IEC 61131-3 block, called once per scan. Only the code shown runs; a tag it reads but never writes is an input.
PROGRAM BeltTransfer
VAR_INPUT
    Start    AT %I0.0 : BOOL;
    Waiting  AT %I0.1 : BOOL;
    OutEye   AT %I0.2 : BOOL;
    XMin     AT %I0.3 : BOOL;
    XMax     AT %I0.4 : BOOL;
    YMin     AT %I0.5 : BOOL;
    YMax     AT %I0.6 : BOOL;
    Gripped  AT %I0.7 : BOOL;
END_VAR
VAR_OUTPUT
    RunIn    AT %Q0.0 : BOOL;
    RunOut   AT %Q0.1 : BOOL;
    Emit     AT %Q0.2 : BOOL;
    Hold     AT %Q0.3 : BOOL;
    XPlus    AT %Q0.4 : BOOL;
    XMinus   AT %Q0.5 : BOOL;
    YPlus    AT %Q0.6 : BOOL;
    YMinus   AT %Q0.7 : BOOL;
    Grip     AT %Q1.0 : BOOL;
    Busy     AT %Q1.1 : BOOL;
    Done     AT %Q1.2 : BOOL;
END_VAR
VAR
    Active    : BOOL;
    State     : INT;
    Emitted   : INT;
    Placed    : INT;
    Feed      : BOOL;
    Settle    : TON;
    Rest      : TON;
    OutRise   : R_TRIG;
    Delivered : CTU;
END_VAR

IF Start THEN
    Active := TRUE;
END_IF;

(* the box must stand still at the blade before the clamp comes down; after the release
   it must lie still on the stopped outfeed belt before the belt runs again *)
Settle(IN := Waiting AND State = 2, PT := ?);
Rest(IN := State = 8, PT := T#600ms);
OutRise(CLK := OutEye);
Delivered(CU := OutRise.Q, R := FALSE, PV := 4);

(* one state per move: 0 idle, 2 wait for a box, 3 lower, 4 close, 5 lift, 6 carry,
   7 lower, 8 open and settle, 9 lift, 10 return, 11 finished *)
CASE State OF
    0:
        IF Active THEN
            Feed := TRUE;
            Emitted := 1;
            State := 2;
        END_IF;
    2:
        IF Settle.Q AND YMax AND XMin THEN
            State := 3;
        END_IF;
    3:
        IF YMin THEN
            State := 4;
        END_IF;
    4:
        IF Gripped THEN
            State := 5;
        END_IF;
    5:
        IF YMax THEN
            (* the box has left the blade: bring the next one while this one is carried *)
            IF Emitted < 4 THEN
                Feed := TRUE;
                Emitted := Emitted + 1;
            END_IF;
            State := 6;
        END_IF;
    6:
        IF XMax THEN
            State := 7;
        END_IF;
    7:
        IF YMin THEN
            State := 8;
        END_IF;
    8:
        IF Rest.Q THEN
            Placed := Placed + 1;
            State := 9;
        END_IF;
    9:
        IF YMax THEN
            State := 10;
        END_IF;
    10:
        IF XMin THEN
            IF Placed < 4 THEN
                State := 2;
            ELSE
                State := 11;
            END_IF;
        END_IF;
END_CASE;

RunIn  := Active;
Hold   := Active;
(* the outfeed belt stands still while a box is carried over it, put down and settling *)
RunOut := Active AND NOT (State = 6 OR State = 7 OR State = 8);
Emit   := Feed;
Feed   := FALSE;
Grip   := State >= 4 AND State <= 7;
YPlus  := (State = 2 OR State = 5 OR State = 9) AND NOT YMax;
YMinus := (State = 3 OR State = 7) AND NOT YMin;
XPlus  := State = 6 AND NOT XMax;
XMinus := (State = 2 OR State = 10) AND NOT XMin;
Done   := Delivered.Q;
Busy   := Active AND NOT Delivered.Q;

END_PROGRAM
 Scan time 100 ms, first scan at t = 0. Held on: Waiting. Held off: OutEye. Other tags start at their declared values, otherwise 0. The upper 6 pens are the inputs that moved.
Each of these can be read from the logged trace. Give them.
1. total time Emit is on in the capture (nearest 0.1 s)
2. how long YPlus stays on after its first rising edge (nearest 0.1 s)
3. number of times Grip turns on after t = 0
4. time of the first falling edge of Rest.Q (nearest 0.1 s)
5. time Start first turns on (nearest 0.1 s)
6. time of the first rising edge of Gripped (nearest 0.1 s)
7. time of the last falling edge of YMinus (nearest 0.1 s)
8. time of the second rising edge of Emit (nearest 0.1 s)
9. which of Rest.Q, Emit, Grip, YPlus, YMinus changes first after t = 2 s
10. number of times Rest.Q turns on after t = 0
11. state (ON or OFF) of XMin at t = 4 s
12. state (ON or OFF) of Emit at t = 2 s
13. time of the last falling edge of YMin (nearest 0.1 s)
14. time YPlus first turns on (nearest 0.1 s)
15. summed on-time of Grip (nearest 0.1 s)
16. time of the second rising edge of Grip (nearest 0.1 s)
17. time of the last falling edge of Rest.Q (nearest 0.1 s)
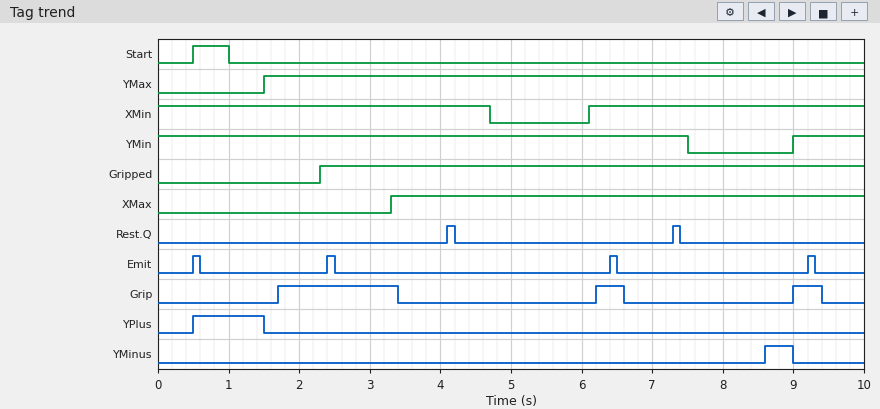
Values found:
0.4 s
1.0 s
3
4.2 s
0.5 s
2.3 s
9.0 s
2.4 s
Emit
2
ON
OFF
7.5 s
0.5 s
2.5 s
6.2 s
7.4 s
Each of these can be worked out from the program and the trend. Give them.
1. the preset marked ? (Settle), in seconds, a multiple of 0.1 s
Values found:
1.0 s
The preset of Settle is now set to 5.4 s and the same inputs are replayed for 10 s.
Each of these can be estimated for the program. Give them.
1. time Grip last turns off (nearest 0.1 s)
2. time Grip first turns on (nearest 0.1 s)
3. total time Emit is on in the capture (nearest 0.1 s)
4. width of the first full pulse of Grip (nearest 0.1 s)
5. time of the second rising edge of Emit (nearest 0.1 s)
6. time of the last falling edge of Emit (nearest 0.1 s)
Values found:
6.6 s
6.2 s
0.2 s
0.4 s
6.4 s
6.5 s
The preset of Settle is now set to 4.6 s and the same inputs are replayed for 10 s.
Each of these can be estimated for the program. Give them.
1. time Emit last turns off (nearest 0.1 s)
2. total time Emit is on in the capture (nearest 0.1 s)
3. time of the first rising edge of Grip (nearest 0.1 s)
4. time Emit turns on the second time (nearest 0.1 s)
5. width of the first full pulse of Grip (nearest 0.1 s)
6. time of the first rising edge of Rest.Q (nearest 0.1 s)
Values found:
6.5 s
0.2 s
6.2 s
6.4 s
0.4 s
7.3 s
